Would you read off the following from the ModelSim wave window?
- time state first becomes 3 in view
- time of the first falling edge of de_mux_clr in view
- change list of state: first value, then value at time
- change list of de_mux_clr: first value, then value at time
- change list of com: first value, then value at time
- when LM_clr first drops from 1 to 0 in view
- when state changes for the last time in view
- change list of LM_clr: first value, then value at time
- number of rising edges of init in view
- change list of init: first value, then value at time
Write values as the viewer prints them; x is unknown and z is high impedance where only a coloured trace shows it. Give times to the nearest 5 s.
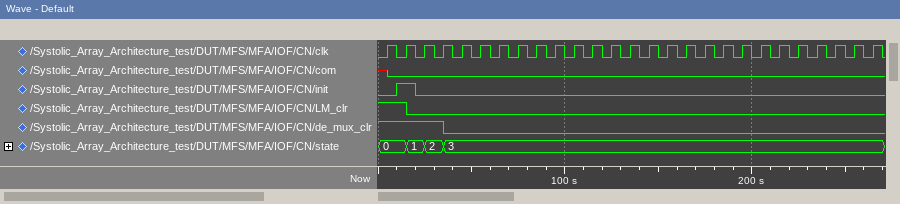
35 s
35 s
0, 1 at 15 s, 2 at 25 s, 3 at 35 s
1, 0 at 35 s
x, 0 at 5 s
15 s
35 s
1, 0 at 15 s
1
0, 1 at 10 s, 0 at 20 s
